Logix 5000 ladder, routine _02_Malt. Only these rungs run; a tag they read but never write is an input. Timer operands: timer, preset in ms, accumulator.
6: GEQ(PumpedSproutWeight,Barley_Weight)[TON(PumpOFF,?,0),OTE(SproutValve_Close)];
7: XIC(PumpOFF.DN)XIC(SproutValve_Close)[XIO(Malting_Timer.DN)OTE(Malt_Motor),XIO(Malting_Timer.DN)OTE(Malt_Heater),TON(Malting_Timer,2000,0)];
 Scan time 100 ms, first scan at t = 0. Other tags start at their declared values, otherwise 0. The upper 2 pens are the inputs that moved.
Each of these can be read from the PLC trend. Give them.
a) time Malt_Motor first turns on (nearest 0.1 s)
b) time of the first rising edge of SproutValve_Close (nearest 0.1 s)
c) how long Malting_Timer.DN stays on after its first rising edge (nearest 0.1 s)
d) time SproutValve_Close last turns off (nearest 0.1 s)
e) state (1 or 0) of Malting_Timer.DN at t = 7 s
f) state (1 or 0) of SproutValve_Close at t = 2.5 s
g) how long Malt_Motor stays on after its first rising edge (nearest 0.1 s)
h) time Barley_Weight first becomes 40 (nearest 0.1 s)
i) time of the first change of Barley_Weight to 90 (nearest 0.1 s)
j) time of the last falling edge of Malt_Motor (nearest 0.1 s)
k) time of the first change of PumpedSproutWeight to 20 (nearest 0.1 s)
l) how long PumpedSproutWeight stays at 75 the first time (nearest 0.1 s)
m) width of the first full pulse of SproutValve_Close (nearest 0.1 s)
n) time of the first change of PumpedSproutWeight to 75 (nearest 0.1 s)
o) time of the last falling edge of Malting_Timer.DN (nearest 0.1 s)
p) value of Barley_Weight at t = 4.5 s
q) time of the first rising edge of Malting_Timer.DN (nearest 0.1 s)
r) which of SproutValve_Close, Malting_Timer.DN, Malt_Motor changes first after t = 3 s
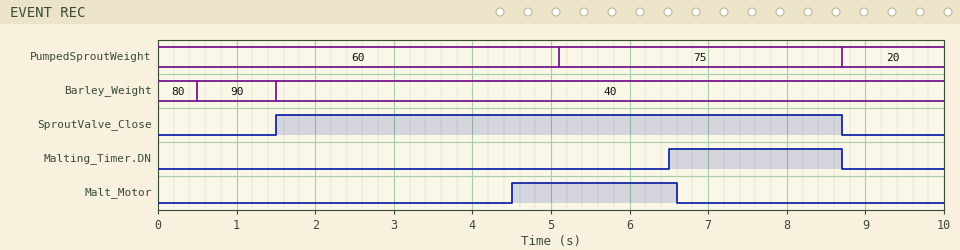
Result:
4.5 s
1.5 s
2.2 s
8.7 s
1
1
2.1 s
1.5 s
0.5 s
6.6 s
8.7 s
3.6 s
7.2 s
5.1 s
8.7 s
40
6.5 s
Malt_Motor
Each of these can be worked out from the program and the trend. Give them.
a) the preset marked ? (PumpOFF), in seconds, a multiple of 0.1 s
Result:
3.0 s
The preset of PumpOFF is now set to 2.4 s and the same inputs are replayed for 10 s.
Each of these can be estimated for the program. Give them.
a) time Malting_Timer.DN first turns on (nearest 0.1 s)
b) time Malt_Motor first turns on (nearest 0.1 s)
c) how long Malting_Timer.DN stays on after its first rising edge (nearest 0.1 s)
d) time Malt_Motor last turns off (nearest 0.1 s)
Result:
5.9 s
3.9 s
2.8 s
6.0 s
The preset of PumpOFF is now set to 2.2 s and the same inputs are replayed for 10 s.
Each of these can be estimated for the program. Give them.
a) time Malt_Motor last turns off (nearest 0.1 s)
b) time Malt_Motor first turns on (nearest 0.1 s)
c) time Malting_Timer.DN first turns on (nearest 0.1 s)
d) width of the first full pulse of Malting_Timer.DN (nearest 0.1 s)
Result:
5.8 s
3.7 s
5.7 s
3.0 s
